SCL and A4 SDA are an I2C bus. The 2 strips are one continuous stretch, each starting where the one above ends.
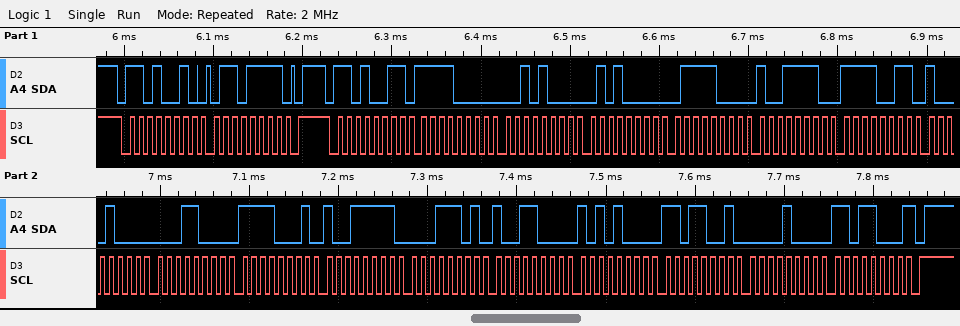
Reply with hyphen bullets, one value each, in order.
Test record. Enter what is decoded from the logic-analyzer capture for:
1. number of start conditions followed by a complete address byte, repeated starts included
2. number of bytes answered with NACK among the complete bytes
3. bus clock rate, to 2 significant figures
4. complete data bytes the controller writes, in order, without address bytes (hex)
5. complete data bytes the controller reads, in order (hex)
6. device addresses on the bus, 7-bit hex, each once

- 2
- 1
- 100 kHz
- 6F
- F0 28 50 78 9E F3 88 18 F1 9F 1D 98 A8 D9 08 D8
- 0x69
